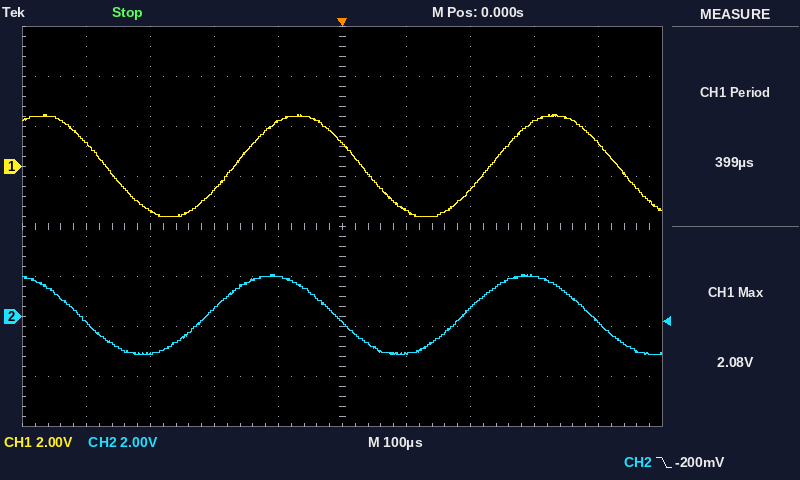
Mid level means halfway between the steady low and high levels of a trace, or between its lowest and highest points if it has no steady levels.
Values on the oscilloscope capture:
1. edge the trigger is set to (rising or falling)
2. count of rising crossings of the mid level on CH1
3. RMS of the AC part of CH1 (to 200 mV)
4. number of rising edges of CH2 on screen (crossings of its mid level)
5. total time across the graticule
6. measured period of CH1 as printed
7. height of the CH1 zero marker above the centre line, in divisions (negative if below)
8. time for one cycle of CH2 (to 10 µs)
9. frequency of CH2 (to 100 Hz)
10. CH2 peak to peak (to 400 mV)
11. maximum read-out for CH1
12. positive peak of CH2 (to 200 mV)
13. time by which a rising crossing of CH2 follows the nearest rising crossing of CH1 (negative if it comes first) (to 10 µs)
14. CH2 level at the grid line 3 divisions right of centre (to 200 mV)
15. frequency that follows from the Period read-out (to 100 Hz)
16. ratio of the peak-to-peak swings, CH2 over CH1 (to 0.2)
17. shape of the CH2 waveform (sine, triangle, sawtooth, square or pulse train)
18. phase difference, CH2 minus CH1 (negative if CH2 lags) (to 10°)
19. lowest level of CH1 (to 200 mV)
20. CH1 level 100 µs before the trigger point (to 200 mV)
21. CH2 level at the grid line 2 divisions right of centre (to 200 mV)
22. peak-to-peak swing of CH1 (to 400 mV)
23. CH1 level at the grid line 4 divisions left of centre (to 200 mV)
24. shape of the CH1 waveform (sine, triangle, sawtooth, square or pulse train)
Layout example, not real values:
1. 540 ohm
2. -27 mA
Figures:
1. falling
2. 2
3. 1.4 V
4. 2
5. 1 ms
6. 399 µs
7. +1.2 div
8. 400 µs
9. 2.5 kHz
10. 3.2 V
11. 2.08 V
12. 1.6 V
13. -40 µs
14. 1.6 V
15. 2.5 kHz
16. 0.8
17. sine
18. +40°
19. -2.0 V
20. 1.8 V
21. 400 mV
22. 4.0 V
23. 1.0 V
24. sine
